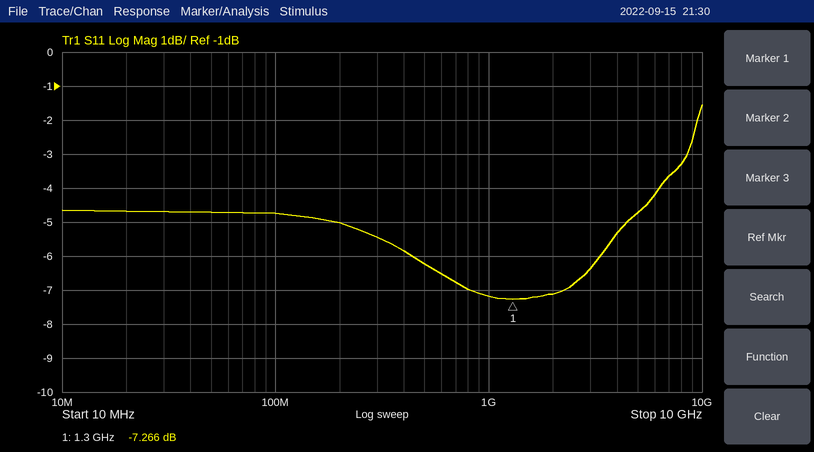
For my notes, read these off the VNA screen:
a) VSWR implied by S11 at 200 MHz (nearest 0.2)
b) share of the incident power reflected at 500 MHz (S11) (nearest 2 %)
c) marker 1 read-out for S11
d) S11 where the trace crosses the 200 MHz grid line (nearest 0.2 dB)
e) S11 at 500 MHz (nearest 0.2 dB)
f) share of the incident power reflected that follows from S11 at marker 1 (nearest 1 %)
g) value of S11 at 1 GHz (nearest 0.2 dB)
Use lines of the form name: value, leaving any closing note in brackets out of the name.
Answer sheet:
VSWR implied by S11 at 200 MHz: 3.6
share of the incident power reflected at 500 MHz (S11): 24 %
marker 1 read-out for S11: -7.266 dB
S11 where the trace crosses the 200 MHz grid line: -5.0 dB
S11 at 500 MHz: -6.2 dB
share of the incident power reflected that follows from S11 at marker 1: 19 %
value of S11 at 1 GHz: -7.2 dB
